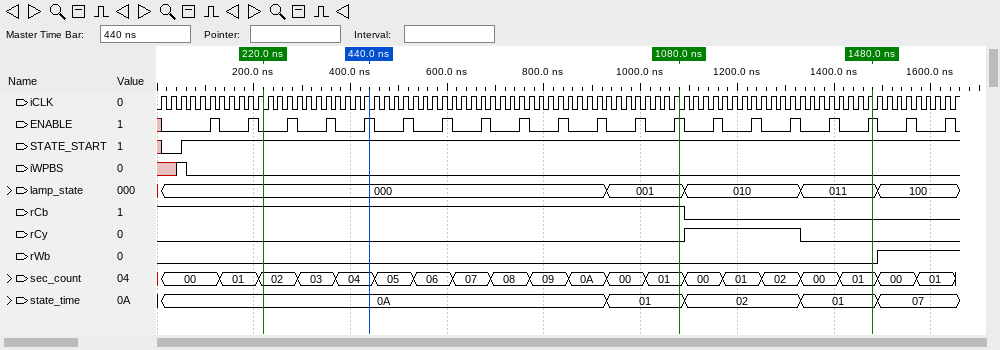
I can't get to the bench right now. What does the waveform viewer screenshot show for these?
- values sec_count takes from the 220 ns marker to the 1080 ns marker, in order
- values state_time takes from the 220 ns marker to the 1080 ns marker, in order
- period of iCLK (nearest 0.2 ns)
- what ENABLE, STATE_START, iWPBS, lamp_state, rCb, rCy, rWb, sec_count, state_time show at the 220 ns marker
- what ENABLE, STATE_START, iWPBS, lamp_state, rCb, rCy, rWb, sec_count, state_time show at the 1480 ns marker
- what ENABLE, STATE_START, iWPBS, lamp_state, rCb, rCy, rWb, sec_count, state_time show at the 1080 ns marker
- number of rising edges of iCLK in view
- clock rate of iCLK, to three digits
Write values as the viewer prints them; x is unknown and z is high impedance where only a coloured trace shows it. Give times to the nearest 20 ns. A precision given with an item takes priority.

02, 03, 04, 05, 06, 07, 08, 09, 0A, 00, 01
0A, 01
20 ns
ENABLE=0, STATE_START=1, iWPBS=0, lamp_state=000, rCb=1, rCy=0, rWb=0, sec_count=02, state_time=0A
ENABLE=1, STATE_START=1, iWPBS=0, lamp_state=011, rCb=0, rCy=0, rWb=0, sec_count=01, state_time=01
ENABLE=1, STATE_START=1, iWPBS=0, lamp_state=001, rCb=1, rCy=0, rWb=0, sec_count=01, state_time=01
83
50.0 MHz
